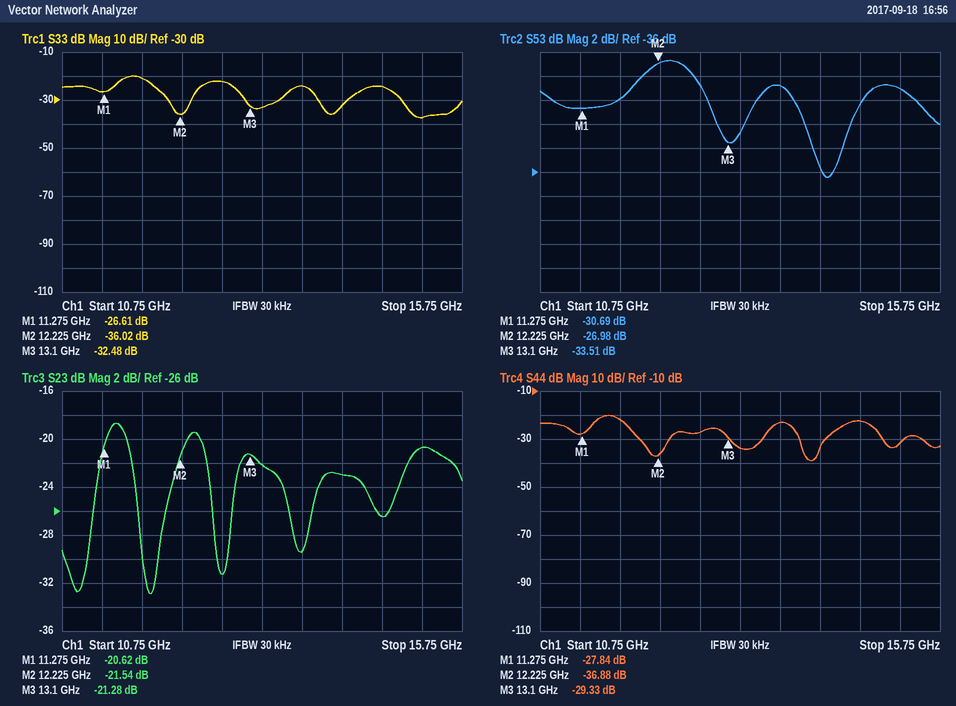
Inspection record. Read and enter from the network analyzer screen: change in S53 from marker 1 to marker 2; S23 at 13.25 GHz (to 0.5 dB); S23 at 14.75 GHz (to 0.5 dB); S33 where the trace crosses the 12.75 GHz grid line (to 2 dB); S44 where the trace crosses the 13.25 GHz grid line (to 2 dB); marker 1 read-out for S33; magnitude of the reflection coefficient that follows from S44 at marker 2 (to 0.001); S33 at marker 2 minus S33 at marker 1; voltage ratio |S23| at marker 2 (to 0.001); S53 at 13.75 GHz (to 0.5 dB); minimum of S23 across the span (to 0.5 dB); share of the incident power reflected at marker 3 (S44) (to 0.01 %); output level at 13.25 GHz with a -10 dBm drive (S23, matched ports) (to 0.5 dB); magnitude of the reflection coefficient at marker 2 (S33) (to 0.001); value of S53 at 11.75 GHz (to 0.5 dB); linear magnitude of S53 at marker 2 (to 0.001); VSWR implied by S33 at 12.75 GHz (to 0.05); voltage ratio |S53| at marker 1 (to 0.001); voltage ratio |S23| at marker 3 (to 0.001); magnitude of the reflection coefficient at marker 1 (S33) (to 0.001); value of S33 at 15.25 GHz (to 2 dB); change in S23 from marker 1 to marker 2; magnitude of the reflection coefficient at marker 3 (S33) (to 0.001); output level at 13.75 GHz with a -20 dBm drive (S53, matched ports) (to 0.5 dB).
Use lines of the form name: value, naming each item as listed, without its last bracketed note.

change in S53 from marker 1 to marker 2: 3.71 dB
S23 at 13.25 GHz: -22.0 dB
S23 at 14.75 GHz: -26.5 dB
S33 where the trace crosses the 12.75 GHz grid line: -22 dB
S44 where the trace crosses the 13.25 GHz grid line: -34 dB
marker 1 read-out for S33: -26.61 dB
magnitude of the reflection coefficient that follows from S44 at marker 2: 0.014
S33 at marker 2 minus S33 at marker 1: -9.41 dB
voltage ratio |S23| at marker 2: 0.084
S53 at 13.75 GHz: -29.0 dB
minimum of S23 across the span: -33.0 dB
share of the incident power reflected at marker 3 (S44): 0.12 %
output level at 13.25 GHz with a -10 dBm drive (S23, matched ports): -32.0 dBm
magnitude of the reflection coefficient at marker 2 (S33): 0.016
value of S53 at 11.75 GHz: -30.0 dB
linear magnitude of S53 at marker 2: 0.045
VSWR implied by S33 at 12.75 GHz: 1.15
voltage ratio |S53| at marker 1: 0.029
voltage ratio |S23| at marker 3: 0.086
magnitude of the reflection coefficient at marker 1 (S33): 0.047
value of S33 at 15.25 GHz: -38 dB
change in S23 from marker 1 to marker 2: -0.92 dB
magnitude of the reflection coefficient at marker 3 (S33): 0.024
output level at 13.75 GHz with a -20 dBm drive (S53, matched ports): -49.0 dBm
